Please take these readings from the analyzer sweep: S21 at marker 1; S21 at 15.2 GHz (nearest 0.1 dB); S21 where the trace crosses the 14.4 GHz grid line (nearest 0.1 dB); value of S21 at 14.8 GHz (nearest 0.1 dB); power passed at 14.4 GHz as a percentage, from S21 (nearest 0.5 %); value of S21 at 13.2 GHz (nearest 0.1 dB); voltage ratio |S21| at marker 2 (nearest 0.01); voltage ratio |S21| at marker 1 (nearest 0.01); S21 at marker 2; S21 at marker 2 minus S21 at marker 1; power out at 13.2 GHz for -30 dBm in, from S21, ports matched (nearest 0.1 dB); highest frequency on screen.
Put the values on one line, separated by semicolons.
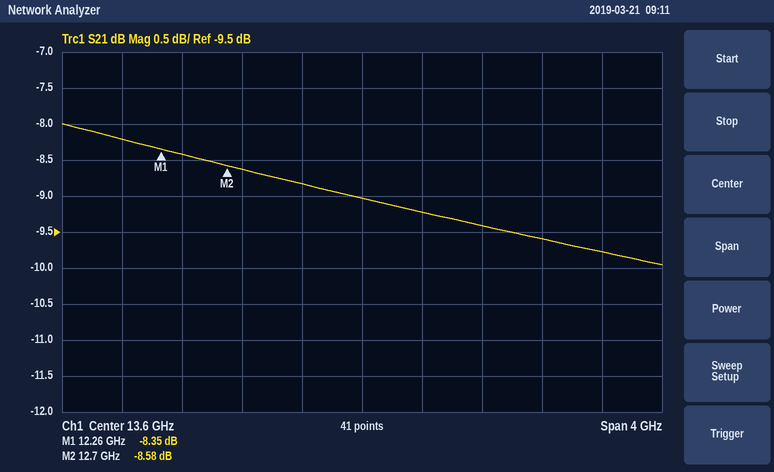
-8.35 dB; -9.8 dB; -9.4 dB; -9.6 dB; 11.5 %; -8.8 dB; 0.37; 0.38; -8.58 dB; -0.23 dB; -38.8 dBm; 15.6 GHz
